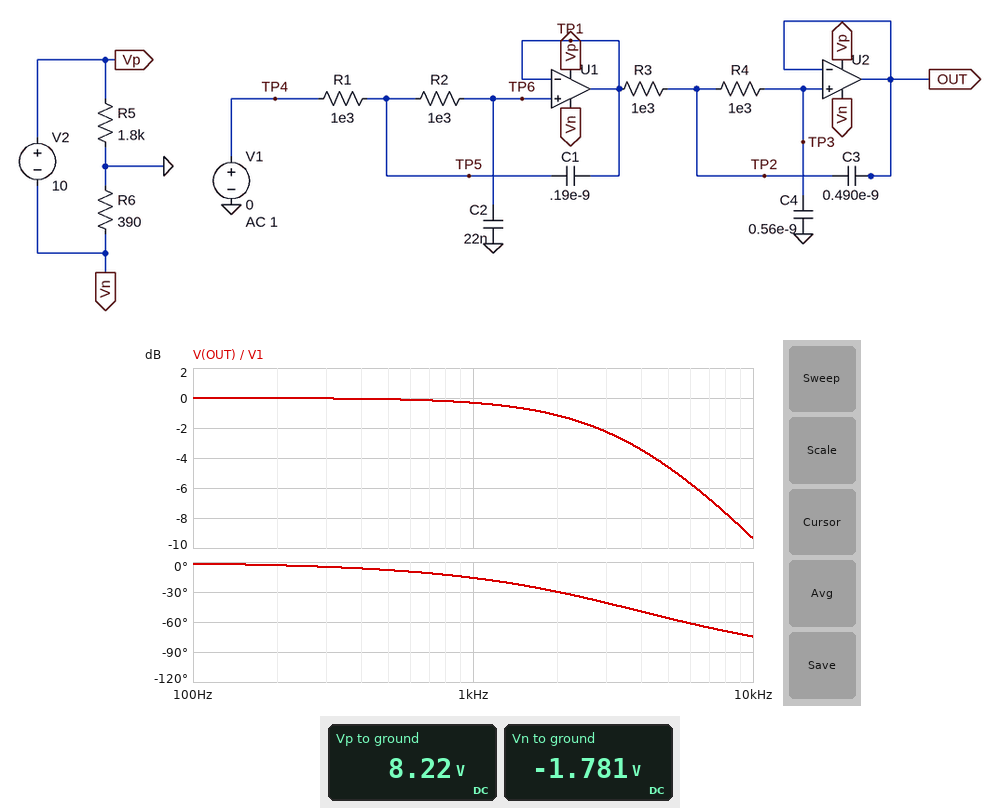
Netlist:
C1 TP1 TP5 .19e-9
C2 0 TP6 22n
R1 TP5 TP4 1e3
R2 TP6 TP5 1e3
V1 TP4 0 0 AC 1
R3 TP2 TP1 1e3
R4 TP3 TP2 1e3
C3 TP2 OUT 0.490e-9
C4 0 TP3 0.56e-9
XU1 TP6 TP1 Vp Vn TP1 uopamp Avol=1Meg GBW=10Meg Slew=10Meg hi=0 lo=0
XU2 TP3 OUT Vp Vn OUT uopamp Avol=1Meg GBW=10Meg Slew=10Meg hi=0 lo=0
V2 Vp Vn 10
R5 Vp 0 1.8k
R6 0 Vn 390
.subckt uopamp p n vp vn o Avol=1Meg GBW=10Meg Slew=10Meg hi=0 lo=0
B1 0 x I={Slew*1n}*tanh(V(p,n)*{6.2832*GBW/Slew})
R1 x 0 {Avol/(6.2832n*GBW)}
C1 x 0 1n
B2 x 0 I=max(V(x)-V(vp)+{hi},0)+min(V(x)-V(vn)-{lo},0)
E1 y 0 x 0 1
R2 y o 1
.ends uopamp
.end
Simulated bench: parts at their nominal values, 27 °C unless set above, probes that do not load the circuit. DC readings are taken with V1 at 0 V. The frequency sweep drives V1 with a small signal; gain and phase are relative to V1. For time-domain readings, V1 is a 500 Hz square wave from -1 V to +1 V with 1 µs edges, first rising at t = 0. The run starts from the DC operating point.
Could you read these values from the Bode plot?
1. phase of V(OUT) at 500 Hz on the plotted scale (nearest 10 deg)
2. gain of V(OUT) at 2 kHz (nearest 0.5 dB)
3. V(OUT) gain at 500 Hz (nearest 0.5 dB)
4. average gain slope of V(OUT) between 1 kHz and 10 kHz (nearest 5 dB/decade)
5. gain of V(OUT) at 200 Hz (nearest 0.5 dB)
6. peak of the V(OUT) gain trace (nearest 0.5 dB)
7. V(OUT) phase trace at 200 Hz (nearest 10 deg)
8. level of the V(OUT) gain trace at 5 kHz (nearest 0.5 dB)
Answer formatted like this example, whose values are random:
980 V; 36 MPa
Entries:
-10 deg; -1.0 dB; 0 dB; -10 dB/decade; 0 dB; 0 dB; 0 deg; -4.5 dB
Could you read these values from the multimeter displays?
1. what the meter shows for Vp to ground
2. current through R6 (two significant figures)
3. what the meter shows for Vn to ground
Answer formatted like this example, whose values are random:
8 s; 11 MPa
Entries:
8.22 V; 4.6 mA; -1.781 V
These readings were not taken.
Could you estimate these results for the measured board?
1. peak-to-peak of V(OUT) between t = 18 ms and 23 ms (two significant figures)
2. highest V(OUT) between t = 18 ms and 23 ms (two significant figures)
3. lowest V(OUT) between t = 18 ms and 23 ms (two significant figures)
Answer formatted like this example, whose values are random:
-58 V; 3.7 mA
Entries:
2.0 V; 1.0 V; -1.0 V
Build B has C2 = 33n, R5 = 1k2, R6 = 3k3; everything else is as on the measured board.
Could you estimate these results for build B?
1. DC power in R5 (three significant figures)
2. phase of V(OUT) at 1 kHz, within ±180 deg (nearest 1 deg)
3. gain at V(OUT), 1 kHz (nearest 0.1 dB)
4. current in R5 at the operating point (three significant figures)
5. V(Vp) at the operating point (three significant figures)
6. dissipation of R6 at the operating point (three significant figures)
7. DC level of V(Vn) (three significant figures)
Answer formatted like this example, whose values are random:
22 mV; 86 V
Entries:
5.93 mW; -23 deg; -0.7 dB; 2.22 mA; 2.67 V; 16.3 mW; -7.33 V
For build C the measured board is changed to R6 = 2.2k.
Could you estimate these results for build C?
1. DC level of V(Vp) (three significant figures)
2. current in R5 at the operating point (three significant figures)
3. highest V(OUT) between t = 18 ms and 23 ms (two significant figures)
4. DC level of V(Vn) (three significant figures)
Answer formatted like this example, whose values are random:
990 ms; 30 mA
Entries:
4.50 V; 2.50 mA; 1.0 V; -5.50 V
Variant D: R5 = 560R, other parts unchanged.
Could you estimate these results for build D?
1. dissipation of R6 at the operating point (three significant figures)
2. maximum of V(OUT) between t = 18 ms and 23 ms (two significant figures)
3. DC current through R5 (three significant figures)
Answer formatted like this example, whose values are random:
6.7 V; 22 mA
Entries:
43.2 mW; 1.0 V; 10.5 mA
